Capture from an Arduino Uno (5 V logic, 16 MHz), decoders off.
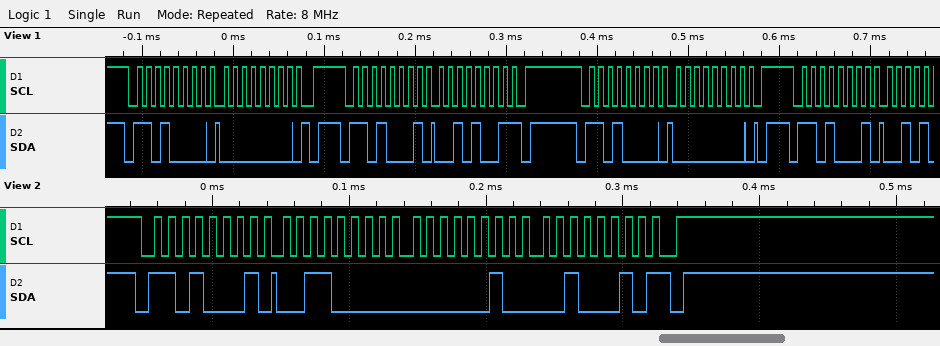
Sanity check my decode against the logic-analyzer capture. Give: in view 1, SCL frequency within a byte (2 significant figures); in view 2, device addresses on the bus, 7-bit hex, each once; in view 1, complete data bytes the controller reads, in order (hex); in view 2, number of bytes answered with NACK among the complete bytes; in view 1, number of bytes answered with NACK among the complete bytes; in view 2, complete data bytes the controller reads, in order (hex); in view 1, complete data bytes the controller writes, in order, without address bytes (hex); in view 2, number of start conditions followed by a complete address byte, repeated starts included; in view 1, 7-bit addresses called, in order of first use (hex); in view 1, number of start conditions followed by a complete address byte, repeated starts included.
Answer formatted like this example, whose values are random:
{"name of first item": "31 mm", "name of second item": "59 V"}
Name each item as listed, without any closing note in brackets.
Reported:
{"in view 1, SCL frequency within a byte": "100 kHz", "in view 2, device addresses on the bus, 7-bit hex, each once": "0x68", "in view 1, complete data bytes the controller reads, in order": "29", "in view 2, number of bytes answered with NACK among the complete bytes": "1", "in view 1, number of bytes answered with NACK among the complete bytes": "1", "in view 2, complete data bytes the controller reads, in order": "30 02 22", "in view 1, complete data bytes the controller writes, in order, without address bytes": "00 00", "in view 2, number of start conditions followed by a complete address byte, repeated starts included": "1", "in view 1, 7-bit addresses called, in order of first use": "0x68", "in view 1, number of start conditions followed by a complete address byte, repeated starts included": "4"}
